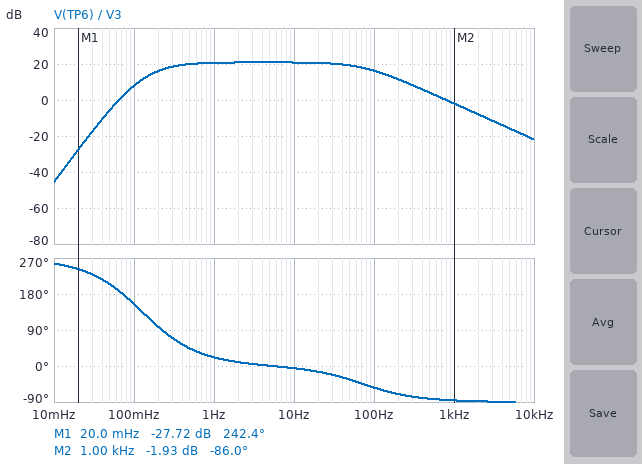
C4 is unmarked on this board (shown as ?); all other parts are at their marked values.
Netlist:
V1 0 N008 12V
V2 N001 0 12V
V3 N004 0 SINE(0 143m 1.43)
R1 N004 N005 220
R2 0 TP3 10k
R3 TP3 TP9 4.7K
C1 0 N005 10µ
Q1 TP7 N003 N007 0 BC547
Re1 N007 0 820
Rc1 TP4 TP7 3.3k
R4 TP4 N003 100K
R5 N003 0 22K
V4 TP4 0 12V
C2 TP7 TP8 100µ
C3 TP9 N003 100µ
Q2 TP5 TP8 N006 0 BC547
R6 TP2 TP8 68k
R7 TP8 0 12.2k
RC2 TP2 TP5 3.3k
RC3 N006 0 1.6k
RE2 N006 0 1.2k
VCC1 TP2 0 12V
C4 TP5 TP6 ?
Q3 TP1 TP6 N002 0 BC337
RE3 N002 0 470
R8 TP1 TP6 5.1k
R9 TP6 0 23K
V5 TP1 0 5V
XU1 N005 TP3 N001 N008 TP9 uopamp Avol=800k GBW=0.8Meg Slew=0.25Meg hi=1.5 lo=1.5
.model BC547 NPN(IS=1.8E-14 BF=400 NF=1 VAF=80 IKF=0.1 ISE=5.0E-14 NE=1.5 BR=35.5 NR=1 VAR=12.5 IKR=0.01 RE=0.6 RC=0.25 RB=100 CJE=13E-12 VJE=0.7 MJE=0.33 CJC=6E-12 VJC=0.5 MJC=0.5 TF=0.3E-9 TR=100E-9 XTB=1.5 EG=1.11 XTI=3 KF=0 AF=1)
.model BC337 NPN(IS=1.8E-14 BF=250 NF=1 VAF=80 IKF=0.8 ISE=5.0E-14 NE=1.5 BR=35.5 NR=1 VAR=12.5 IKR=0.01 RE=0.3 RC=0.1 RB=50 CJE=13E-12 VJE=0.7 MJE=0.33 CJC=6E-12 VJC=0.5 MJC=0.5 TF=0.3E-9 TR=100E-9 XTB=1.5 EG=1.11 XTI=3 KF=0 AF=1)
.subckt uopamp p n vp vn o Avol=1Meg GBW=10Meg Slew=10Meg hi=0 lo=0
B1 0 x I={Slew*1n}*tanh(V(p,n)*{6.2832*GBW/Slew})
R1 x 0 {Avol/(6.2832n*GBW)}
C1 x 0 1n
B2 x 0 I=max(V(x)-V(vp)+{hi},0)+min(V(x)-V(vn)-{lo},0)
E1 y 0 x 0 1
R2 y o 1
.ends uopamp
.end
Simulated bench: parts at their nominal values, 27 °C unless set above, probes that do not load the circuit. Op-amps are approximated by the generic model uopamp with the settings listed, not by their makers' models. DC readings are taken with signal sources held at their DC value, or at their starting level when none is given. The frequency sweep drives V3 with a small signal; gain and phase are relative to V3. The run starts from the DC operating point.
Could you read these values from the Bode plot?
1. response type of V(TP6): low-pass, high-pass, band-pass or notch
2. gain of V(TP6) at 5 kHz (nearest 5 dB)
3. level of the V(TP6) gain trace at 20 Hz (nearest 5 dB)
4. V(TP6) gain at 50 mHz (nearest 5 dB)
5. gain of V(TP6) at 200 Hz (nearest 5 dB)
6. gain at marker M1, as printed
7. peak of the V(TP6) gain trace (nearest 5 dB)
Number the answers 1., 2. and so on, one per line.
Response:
1. band-pass
2. -15 dB
3. 20 dB
4. -5 dB
5. 10 dB
6. -27.72 dB
7. 20 dB
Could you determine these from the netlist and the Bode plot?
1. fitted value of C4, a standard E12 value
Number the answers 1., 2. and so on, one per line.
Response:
1. 120 µF
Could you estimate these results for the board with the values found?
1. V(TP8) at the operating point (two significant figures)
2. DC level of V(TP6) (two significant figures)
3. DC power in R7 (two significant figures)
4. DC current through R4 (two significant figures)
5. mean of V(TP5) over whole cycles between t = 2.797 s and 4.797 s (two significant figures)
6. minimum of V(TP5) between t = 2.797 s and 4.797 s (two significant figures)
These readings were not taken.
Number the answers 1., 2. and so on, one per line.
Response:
1. 1.8 V
2. 4.0 V
3. 260 µW
4. 99 µA
5. 6.6 V
6. 5.0 V
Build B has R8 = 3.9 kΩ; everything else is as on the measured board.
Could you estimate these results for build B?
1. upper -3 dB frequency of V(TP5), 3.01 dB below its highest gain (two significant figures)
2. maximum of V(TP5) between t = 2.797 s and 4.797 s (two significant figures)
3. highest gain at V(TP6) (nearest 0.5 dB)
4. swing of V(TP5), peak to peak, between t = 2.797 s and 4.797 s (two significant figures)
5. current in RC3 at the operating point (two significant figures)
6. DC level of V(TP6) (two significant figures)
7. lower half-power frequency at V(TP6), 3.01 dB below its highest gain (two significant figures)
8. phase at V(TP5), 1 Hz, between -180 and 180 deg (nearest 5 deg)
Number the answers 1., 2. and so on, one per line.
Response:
1. 37 Hz
2. 8.1 V
3. 20.0 dB
4. 2.9 V
5. 700 µA
6. 4.2 V
7. 280 mHz
8. 0 deg
